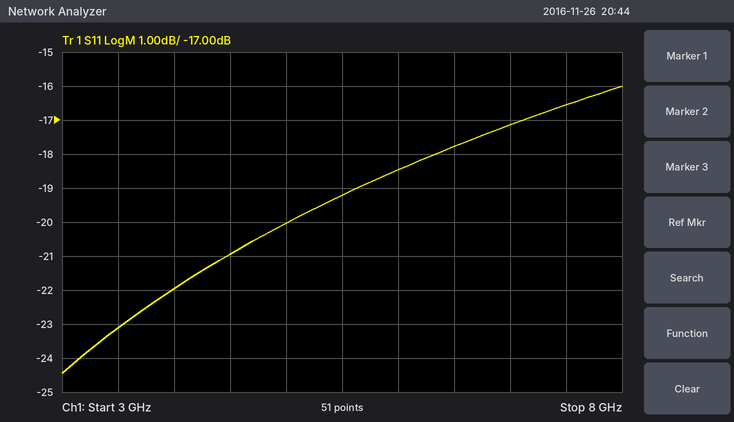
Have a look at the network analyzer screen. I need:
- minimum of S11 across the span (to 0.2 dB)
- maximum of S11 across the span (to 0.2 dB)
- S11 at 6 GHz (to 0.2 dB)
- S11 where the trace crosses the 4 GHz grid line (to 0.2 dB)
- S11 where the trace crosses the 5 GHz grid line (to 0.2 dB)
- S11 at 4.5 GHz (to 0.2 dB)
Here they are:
-24.4 dB
-16.0 dB
-18.4 dB
-22.0 dB
-20.0 dB
-21.0 dB
